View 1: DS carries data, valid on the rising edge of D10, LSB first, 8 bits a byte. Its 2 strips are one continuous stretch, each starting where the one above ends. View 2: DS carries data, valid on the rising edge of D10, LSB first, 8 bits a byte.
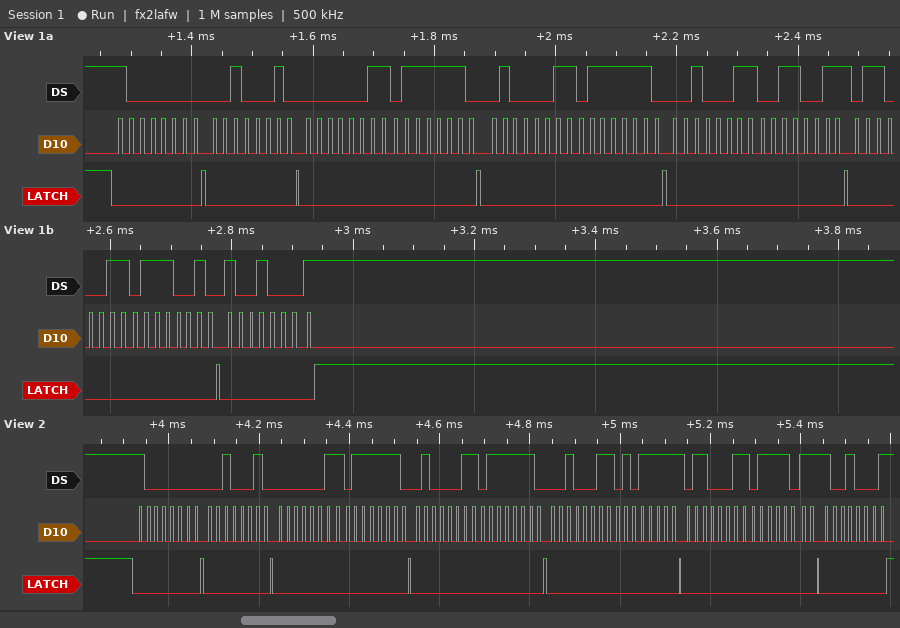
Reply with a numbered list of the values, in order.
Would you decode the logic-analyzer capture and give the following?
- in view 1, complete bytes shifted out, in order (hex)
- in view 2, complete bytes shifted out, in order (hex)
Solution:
1. 01 44 C0 7E C2 7E C4 CC C6 4E 89
2. 01 44 C0 7E C2 7E C4 FA C6 DE 89
